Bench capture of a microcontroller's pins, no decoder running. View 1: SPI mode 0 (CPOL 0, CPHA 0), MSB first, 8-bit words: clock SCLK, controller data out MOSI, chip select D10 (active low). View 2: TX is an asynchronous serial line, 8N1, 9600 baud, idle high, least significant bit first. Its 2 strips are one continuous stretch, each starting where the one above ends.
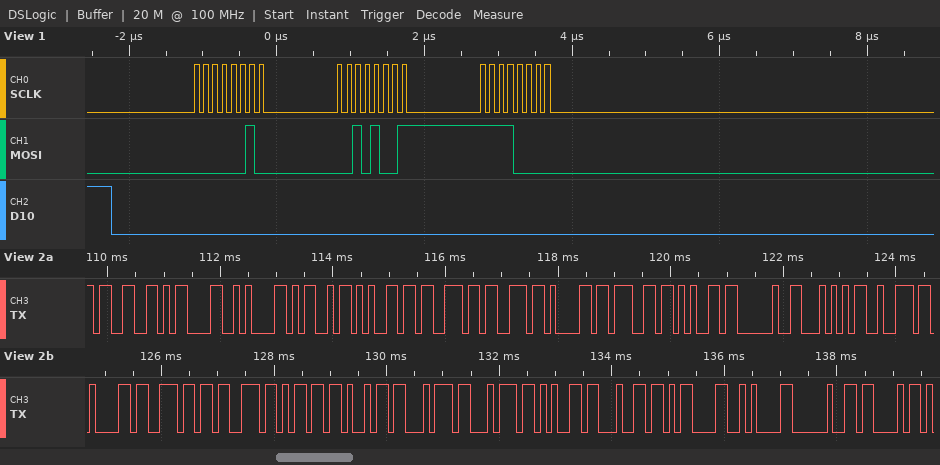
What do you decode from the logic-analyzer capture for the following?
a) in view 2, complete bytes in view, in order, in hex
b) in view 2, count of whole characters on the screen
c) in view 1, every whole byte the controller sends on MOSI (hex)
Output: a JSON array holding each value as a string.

["0x33 0x0D 0x0A 0x4D 0x65 0x73 0x73 0x61 0x67 0x65 0x20 0x54 0x72 0x61 0x6E 0x73 0x6D 0x69 0x74 0x74 0x65 0x64 0x0D 0x0A 0x20 0x43", "26", "02 29 F0"]
